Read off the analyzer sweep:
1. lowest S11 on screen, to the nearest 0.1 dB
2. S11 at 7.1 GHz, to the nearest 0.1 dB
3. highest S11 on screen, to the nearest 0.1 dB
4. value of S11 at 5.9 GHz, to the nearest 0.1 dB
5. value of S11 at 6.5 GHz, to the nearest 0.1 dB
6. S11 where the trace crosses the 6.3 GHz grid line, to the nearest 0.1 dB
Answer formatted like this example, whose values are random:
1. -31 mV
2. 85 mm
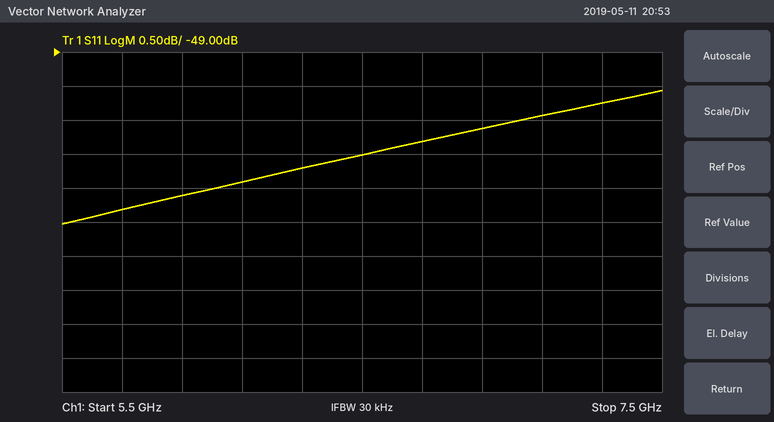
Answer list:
1. -51.5 dB
2. -49.9 dB
3. -49.6 dB
4. -51.1 dB
5. -50.5 dB
6. -50.7 dB
